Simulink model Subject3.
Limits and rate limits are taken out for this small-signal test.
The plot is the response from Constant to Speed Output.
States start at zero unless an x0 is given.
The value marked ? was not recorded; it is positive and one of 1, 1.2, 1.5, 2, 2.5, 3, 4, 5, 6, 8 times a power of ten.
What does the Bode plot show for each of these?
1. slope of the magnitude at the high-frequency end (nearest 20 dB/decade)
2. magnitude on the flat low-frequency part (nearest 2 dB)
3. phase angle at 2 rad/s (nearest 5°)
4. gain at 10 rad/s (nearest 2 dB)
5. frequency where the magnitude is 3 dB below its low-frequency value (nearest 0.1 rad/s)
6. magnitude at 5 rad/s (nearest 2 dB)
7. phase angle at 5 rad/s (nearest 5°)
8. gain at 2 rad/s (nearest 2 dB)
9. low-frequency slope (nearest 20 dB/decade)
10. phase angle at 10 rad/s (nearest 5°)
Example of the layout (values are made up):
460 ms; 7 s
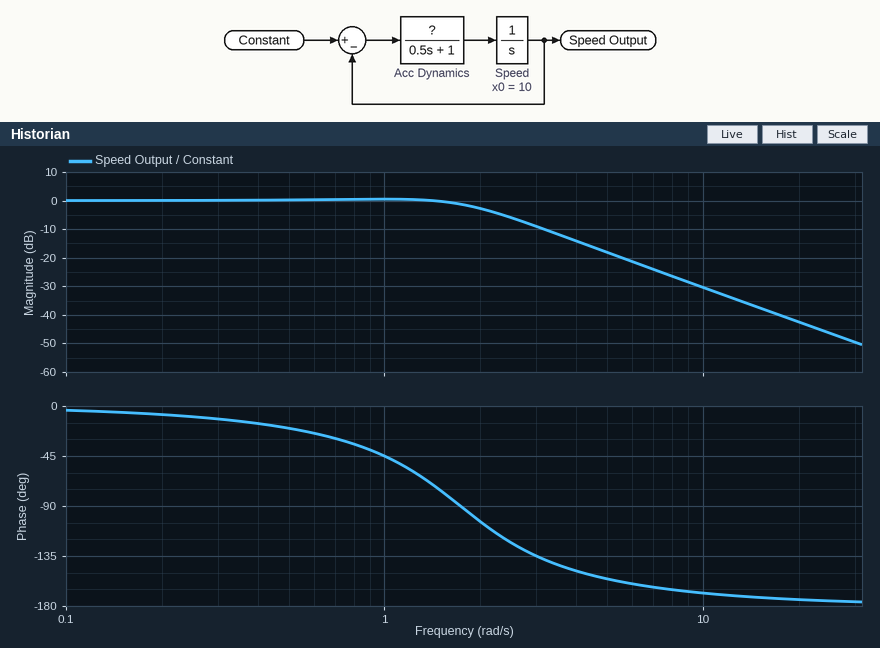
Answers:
-40 dB/decade; 0 dB; -105°; -30 dB; 2.0 rad/s; -18 dB; -155°; -2 dB; 0 dB/decade; -170°
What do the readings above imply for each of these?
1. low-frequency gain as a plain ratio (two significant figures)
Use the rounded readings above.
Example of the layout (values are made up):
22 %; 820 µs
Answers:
1.0
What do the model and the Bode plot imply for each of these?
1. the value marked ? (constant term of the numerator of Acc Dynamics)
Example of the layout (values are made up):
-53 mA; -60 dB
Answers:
1.5
